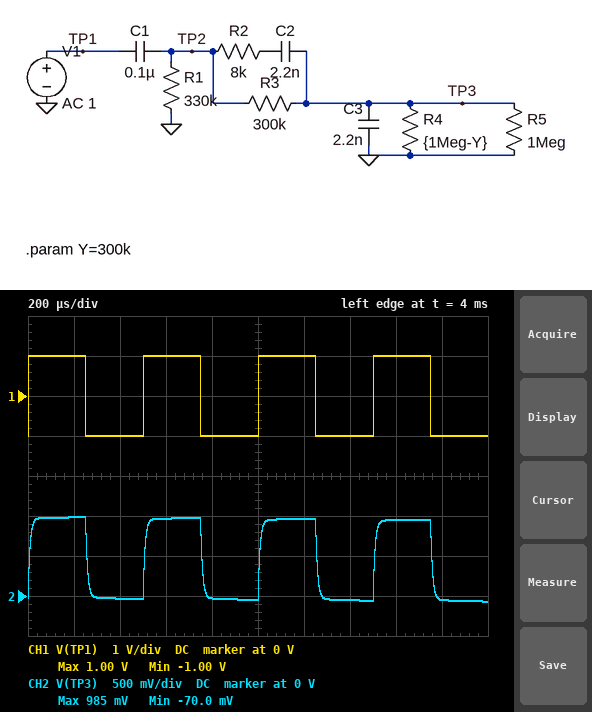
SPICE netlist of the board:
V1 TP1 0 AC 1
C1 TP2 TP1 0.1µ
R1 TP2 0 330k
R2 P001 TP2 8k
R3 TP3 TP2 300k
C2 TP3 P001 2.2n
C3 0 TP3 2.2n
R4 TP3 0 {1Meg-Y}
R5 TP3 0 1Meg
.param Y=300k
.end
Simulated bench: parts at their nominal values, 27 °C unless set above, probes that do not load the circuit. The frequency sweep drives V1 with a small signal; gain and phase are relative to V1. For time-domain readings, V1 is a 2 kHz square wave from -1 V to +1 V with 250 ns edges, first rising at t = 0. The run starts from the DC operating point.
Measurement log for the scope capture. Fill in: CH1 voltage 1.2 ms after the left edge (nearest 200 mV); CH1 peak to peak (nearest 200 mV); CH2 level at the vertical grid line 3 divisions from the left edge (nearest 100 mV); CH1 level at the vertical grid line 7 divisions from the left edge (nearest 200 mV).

1.0 V
2.0 V
1.0 V
-1.0 V
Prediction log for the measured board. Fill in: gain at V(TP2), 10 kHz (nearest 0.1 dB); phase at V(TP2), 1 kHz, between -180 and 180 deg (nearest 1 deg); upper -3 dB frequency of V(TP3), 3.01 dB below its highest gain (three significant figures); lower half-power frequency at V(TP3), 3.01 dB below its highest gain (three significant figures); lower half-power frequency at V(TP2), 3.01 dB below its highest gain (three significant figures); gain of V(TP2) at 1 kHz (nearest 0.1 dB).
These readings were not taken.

-0.1 dB
0 deg
14.2 kHz
6.77 Hz
7.14 Hz
-0.1 dB
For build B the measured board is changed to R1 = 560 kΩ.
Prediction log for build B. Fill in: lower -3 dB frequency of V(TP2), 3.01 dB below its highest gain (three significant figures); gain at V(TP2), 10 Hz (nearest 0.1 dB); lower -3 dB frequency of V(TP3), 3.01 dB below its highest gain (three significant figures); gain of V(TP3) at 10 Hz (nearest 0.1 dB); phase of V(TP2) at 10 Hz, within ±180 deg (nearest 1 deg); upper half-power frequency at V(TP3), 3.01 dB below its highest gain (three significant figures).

5.14 Hz
-1.1 dB
4.91 Hz
-5.8 dB
27 deg
14.0 kHz
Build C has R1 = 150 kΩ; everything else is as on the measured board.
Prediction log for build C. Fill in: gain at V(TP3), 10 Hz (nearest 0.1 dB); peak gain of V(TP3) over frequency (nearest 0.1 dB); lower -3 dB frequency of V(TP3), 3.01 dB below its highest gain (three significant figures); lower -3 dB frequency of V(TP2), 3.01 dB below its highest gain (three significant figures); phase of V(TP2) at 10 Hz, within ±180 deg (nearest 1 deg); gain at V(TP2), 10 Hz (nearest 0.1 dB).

-9.0 dB
-5.1 dB
12.0 Hz
13.0 Hz
52 deg
-4.3 dB
